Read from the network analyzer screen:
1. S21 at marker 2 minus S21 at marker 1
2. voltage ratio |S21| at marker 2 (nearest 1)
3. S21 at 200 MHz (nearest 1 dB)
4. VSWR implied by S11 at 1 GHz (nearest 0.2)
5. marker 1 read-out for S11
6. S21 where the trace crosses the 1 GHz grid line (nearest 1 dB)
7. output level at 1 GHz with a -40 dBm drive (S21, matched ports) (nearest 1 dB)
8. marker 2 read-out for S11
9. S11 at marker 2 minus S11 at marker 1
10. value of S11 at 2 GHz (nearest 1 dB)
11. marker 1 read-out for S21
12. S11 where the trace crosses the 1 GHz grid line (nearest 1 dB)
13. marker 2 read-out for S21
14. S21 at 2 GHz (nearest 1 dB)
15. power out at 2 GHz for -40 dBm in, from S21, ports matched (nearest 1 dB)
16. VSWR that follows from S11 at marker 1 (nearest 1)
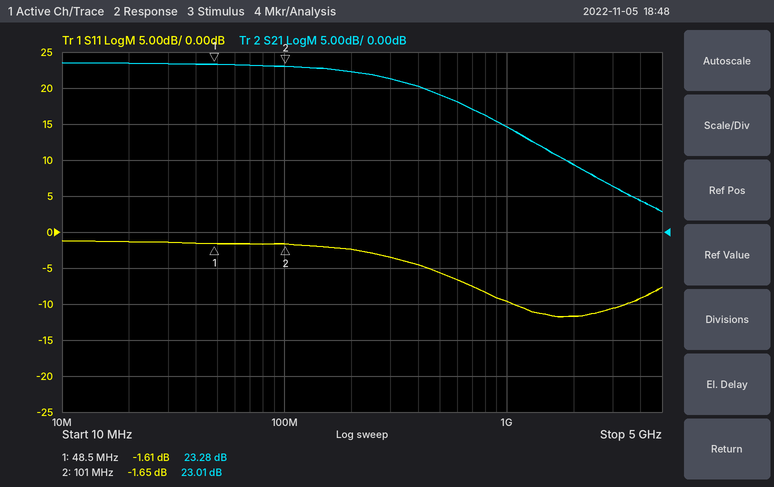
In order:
-0.27 dB
14
22 dB
2.0
-1.61 dB
15 dB
-25 dBm
-1.65 dB
-0.04 dB
-12 dB
23.28 dB
-10 dB
23.01 dB
9 dB
-31 dBm
11
